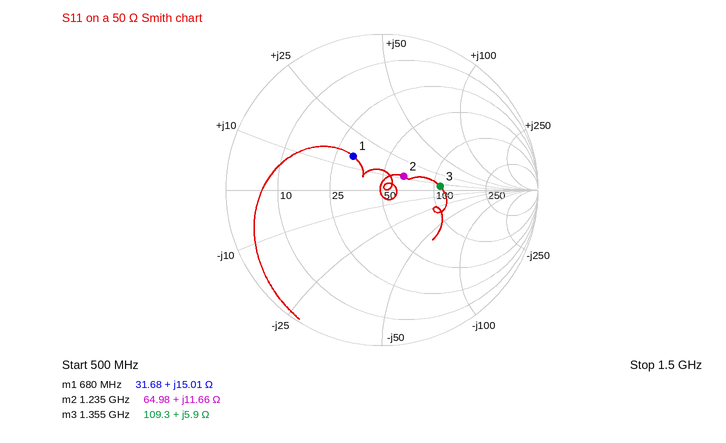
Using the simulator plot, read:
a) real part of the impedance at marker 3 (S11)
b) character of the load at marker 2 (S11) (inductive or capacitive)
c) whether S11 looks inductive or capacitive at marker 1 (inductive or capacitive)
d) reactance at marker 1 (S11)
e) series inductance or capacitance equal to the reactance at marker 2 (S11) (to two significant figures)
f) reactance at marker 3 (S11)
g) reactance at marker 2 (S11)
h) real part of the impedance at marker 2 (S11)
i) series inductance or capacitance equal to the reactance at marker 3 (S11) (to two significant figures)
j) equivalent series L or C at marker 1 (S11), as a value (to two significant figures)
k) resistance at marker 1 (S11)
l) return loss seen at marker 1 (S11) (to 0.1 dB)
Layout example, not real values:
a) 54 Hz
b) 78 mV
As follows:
a) 109.3 Ω
b) inductive
c) inductive
d) +15.01 Ω
e) 1.5 nH
f) +5.9 Ω
g) +11.66 Ω
h) 64.98 Ω
i) 690 pH
j) 3.5 nH
k) 31.68 Ω
l) 10.9 dB
